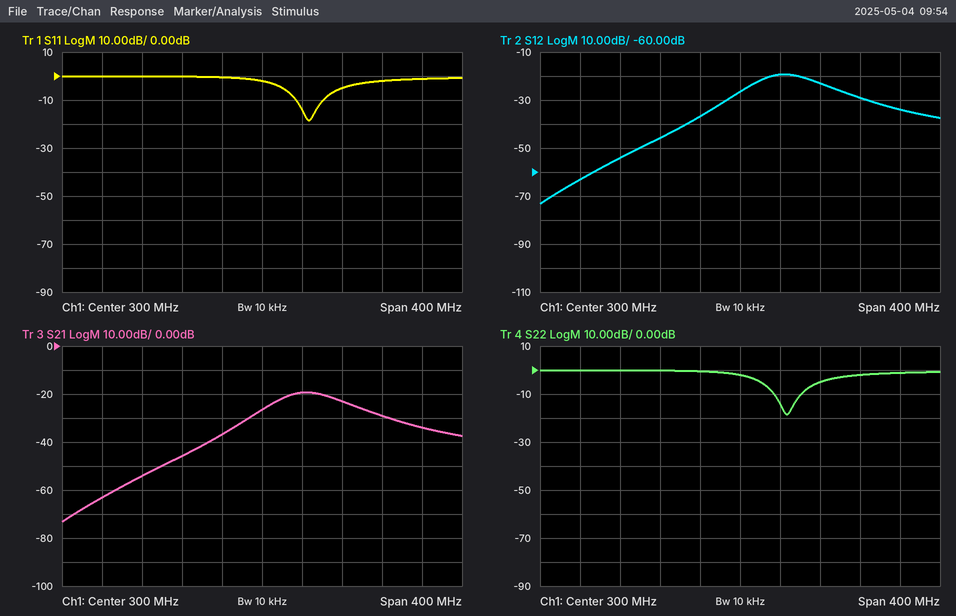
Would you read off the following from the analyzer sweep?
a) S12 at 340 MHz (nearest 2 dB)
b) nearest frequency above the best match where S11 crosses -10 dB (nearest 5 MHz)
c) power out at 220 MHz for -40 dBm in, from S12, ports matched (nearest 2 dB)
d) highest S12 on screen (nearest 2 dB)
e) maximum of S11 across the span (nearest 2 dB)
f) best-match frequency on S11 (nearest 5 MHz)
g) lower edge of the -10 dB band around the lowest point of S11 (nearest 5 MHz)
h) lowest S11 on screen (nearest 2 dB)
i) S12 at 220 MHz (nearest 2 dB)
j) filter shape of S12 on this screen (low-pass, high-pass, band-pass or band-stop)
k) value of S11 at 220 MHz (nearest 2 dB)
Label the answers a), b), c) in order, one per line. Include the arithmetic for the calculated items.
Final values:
a) -20 dB
b) 360 MHz
c) -40 dBm + (-46 dB) = -86 dBm
d) -20 dB
e) 0 dB
f) 345 MHz
g) 335 MHz
h) -18 dB
i) -46 dB
j) band-pass
k) 0 dB
